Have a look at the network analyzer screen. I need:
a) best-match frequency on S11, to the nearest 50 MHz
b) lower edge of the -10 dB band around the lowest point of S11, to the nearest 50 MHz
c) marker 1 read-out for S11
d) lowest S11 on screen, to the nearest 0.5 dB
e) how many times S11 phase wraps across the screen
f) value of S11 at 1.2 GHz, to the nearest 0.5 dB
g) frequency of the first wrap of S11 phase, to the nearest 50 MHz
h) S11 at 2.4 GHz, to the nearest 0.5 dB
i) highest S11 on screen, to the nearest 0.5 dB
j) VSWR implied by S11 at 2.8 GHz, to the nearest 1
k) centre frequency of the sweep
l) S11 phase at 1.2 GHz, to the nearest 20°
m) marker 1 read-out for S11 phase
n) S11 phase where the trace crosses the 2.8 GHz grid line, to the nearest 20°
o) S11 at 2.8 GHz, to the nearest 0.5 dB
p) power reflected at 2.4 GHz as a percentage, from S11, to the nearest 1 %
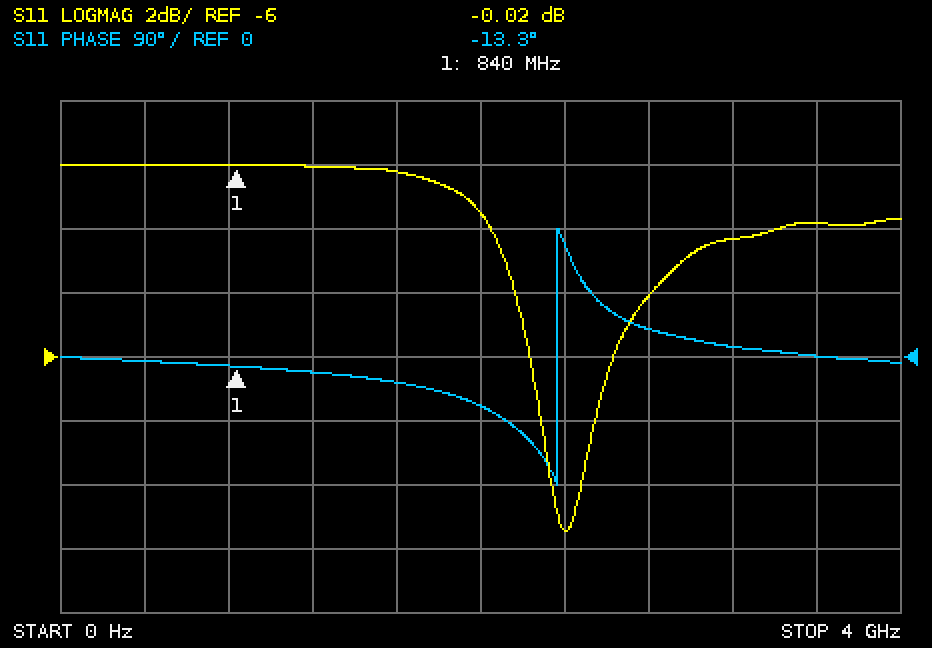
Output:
2.40 GHz
2.35 GHz
-0.02 dB
-11.5 dB
1
0.0 dB
2.35 GHz
-11.5 dB
0.0 dB
4
2 GHz
-20°
-13.3°
40°
-4.0 dB
7 %
